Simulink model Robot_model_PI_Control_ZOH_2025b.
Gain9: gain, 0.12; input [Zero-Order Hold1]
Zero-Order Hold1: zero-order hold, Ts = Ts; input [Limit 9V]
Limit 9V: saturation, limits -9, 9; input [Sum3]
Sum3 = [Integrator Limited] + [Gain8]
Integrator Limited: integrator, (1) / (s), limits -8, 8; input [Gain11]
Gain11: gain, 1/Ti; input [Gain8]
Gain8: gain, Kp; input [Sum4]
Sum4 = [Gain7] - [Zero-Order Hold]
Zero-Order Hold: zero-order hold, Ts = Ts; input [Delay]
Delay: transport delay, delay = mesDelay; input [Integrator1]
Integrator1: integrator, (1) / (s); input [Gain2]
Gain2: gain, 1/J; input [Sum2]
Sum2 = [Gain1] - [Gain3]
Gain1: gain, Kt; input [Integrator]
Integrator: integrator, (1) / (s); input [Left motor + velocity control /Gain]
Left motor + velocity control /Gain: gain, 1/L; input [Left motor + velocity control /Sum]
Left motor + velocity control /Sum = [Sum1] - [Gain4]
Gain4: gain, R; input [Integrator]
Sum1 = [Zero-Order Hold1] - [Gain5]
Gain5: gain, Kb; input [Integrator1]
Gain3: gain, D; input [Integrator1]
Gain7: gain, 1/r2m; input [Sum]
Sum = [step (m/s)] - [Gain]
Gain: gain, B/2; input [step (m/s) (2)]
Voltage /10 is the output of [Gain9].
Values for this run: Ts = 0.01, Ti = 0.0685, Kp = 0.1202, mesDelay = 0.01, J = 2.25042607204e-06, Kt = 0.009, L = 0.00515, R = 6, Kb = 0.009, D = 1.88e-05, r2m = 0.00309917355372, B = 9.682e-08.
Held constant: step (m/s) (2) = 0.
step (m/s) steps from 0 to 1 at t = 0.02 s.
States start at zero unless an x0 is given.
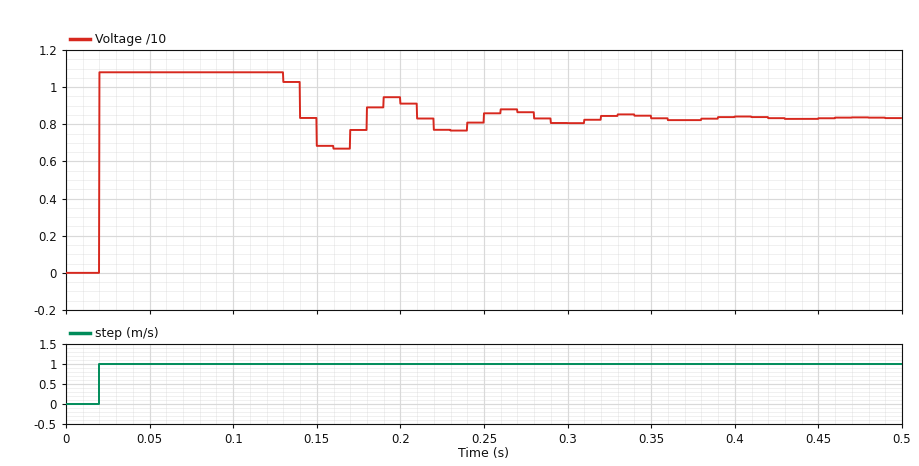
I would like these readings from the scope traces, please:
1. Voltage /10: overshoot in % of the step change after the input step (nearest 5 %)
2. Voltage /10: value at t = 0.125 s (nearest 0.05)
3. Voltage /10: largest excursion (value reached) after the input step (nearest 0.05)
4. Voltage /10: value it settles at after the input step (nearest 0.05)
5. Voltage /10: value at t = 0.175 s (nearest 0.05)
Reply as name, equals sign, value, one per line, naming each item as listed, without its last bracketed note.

Voltage /10: overshoot in % of the step change after the input step = 30 %
Voltage /10: value at t = 0.125 s = 1.10
Voltage /10: largest excursion (value reached) after the input step = 1.10
Voltage /10: value it settles at after the input step = 0.85
Voltage /10: value at t = 0.175 s = 0.75
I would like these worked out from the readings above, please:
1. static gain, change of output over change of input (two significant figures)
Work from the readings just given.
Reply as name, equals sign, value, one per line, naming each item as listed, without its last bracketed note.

static gain, change of output over change of input = 0.85
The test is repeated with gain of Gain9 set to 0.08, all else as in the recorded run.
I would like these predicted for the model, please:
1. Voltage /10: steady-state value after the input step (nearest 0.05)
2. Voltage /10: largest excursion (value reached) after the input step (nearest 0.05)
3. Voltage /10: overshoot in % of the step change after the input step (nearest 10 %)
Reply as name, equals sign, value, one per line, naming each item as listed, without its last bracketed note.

Voltage /10: steady-state value after the input step = 0.55
Voltage /10: largest excursion (value reached) after the input step = 0.70
Voltage /10: overshoot in % of the step change after the input step = 30 %
